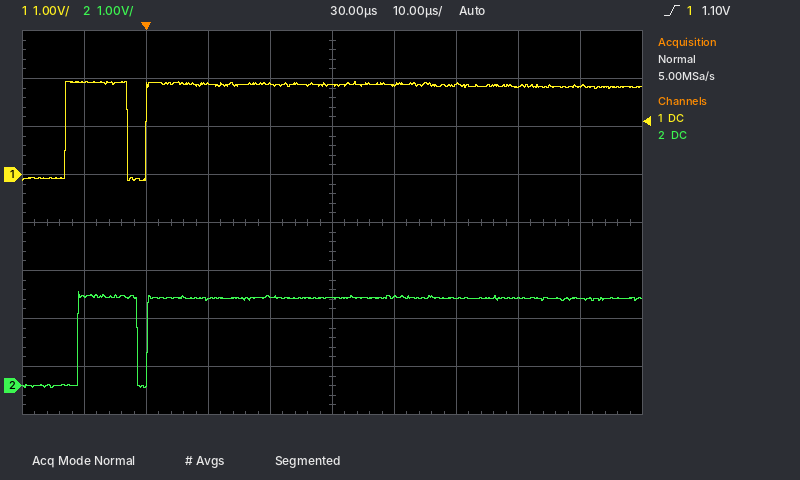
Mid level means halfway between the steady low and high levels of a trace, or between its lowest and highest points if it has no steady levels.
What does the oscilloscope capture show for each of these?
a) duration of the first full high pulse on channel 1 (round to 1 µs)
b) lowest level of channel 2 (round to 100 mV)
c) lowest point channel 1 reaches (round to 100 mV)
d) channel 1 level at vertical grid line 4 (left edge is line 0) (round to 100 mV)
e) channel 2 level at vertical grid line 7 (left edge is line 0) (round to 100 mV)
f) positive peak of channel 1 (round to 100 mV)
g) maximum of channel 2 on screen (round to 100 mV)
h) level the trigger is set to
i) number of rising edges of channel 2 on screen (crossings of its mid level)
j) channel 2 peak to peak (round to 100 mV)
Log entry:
10 µs
0.0 V
-100 mV
1.9 V
1.8 V
1.9 V
2.0 V
1.10 V
2
2.0 V
